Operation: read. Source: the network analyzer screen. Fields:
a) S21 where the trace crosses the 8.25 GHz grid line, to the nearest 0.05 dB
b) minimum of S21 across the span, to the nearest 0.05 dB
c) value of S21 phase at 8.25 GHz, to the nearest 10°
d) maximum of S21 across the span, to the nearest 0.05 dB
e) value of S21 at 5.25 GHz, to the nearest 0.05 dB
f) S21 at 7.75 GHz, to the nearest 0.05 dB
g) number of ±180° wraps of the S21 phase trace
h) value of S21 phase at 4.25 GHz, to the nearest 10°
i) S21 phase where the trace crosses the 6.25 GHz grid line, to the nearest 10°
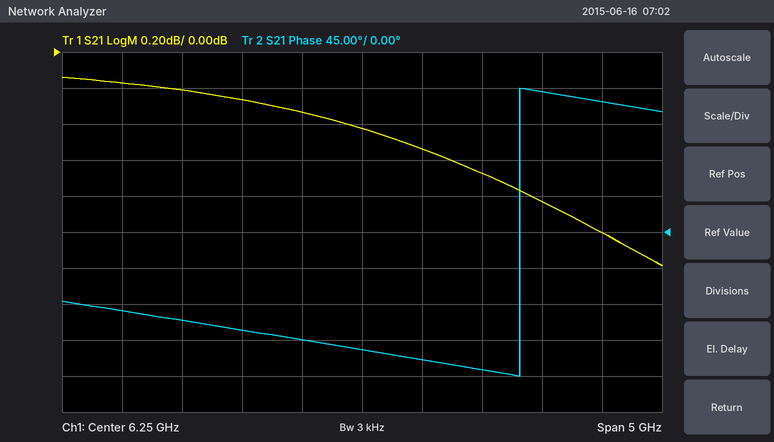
-1.00 dB
-1.20 dB
160°
-0.15 dB
-0.25 dB
-0.85 dB
1
-100°
-150°
